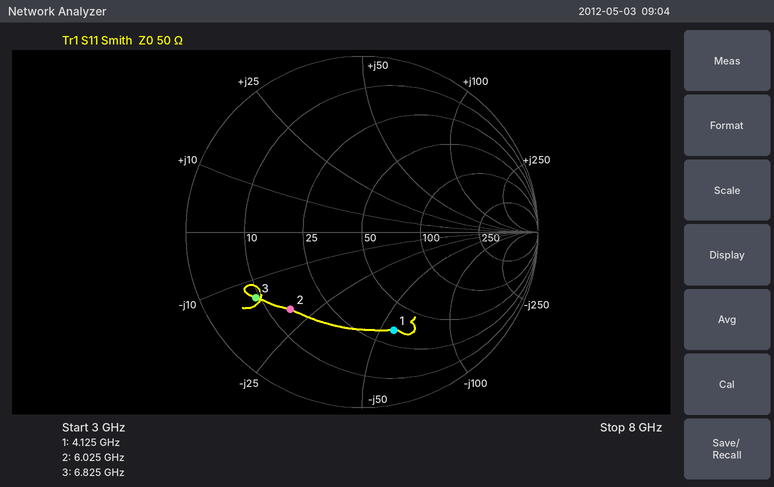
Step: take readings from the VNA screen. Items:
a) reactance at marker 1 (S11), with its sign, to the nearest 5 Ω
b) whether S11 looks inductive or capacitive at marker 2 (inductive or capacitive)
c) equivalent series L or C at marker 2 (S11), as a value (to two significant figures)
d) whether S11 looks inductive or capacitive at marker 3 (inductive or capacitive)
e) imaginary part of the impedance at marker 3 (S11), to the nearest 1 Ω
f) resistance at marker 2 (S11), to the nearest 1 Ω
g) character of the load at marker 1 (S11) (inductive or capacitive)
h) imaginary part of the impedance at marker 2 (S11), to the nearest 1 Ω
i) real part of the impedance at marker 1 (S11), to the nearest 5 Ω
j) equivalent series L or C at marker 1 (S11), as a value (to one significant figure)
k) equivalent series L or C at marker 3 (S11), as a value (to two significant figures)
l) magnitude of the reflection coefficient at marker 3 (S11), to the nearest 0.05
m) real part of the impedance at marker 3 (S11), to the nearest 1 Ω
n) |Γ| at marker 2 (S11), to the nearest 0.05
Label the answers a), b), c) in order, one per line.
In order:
a) -55 Ω
b) capacitive
c) 1.3 pF
d) capacitive
e) -14 Ω
f) 15 Ω
g) capacitive
h) -20 Ω
i) 35 Ω
j) 700 fF
k) 1.7 pF
l) 0.70
m) 9 Ω
n) 0.60
